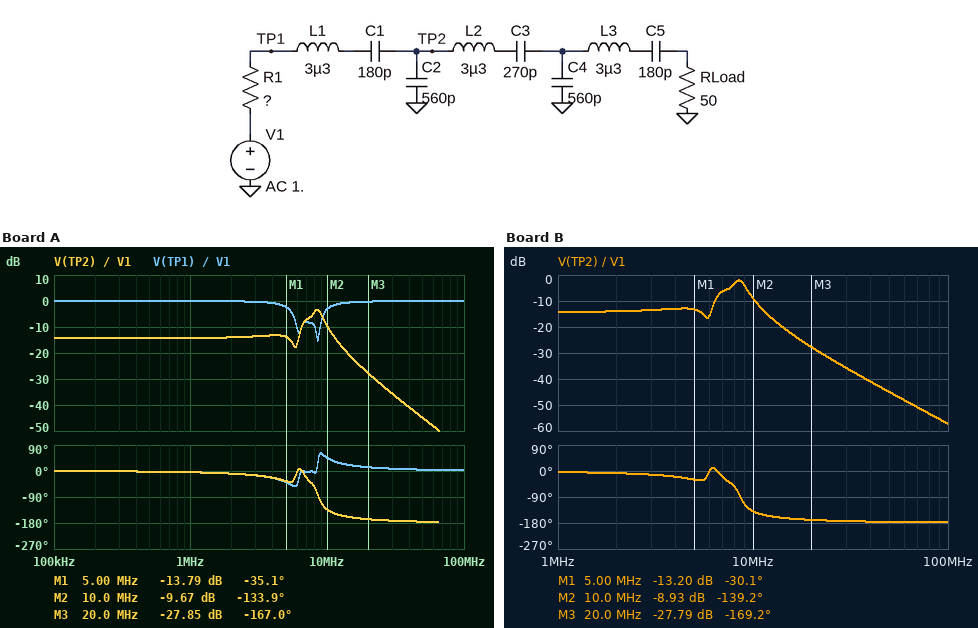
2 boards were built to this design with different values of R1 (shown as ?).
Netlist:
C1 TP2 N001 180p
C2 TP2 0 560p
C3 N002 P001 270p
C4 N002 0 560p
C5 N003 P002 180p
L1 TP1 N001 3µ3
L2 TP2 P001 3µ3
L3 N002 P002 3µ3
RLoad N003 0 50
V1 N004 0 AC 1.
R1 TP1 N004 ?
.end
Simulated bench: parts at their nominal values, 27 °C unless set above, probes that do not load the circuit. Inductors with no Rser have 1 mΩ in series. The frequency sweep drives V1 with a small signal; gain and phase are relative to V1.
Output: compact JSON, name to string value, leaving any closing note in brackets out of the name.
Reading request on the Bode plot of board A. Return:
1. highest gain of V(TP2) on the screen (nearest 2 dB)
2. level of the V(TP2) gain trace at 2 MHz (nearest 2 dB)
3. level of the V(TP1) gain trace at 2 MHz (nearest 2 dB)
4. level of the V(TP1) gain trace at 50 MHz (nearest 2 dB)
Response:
{"highest gain of V(TP2) on the screen": "-4 dB", "level of the V(TP2) gain trace at 2 MHz": "-14 dB", "level of the V(TP1) gain trace at 2 MHz": "0 dB", "level of the V(TP1) gain trace at 50 MHz": "0 dB"}
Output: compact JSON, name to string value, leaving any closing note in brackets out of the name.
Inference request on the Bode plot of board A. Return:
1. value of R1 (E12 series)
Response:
{"value of R1": "82 Ω"}
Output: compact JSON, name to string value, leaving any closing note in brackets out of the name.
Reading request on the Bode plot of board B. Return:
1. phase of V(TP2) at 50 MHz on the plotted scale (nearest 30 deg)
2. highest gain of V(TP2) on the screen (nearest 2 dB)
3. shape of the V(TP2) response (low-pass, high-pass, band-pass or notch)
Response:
{"phase of V(TP2) at 50 MHz on the plotted scale": "-180 deg", "highest gain of V(TP2) on the screen": "-2 dB", "shape of the V(TP2) response": "low-pass"}
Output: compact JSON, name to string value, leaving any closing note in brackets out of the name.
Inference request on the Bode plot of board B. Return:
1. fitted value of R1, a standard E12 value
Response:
{"fitted value of R1, a standard E12 value": "68 Ω"}
